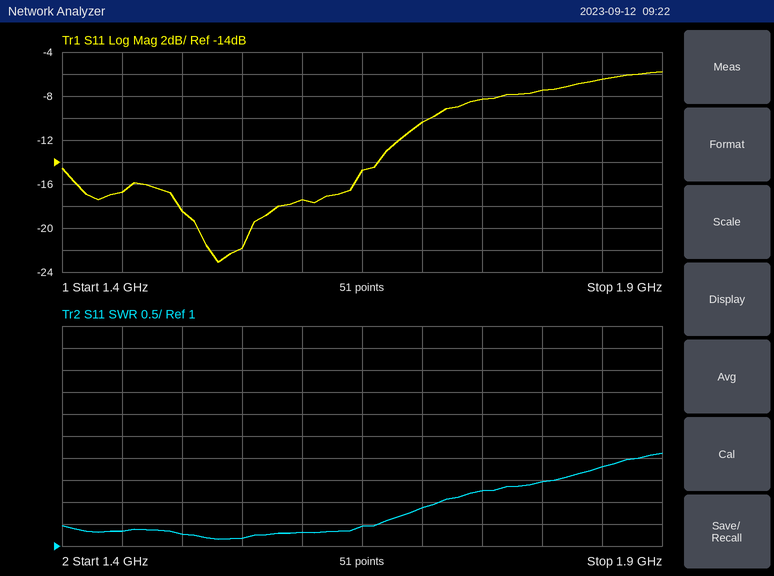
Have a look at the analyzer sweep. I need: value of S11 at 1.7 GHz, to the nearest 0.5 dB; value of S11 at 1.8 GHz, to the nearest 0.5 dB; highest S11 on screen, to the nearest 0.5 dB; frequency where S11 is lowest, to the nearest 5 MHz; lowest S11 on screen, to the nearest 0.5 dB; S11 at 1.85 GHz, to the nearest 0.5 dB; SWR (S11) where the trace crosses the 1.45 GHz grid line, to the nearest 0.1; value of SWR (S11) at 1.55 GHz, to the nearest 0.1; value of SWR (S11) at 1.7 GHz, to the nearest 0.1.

-10.5 dB
-7.5 dB
-6.0 dB
1.530 GHz
-23.0 dB
-6.5 dB
1.3
1.2
1.9
